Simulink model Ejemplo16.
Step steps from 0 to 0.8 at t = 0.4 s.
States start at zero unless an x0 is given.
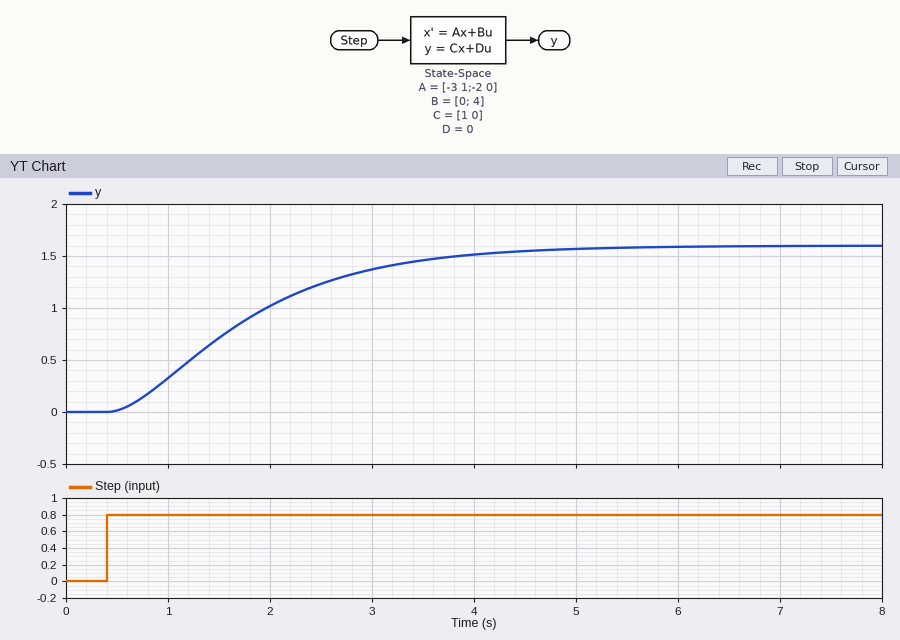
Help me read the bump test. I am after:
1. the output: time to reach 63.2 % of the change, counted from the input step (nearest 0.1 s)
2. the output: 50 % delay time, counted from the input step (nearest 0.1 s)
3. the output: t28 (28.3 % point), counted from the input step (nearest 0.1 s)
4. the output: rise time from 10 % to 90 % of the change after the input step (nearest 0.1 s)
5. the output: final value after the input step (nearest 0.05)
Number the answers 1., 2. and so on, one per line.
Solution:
1. 1.6 s
2. 1.2 s
3. 0.8 s
4. 2.6 s
5. 1.60
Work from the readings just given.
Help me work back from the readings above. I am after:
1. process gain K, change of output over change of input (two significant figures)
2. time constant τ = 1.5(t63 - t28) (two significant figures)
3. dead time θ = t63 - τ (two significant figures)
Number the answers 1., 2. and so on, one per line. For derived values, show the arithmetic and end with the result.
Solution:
1. (1.6 - 0) / 0.8 = 2.0
2. 1.5 × (1.6 - 0.8) = 1.2 s
3. 1.6 - 1.2 = 0.40 s
